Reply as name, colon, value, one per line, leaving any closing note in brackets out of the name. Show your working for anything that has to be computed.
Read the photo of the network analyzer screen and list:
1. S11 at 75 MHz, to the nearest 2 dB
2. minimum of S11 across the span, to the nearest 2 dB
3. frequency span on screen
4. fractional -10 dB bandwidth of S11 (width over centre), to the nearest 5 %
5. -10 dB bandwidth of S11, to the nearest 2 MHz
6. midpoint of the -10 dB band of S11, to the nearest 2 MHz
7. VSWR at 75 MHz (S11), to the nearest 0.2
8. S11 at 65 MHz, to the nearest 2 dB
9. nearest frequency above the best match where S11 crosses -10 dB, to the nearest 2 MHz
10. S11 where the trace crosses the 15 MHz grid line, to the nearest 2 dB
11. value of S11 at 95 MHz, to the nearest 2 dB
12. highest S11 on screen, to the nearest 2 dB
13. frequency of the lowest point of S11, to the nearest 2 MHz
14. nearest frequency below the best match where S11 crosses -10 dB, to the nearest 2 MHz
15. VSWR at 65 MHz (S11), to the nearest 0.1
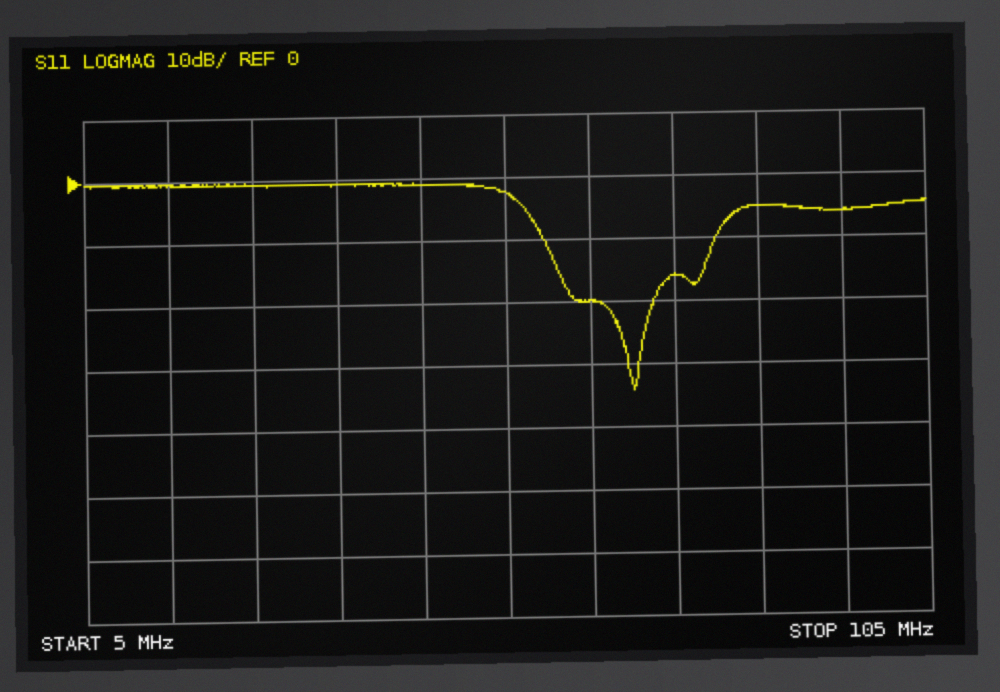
S11 at 75 MHz, to the nearest 2 dB: -16 dB
minimum of S11 across the span, to the nearest 2 dB: -34 dB
frequency span on screen: 100 MHz
fractional -10 dB bandwidth of S11 (width over centre), to the nearest 5 %: 20 MHz / 70 MHz ≈ 28.6 %, so 30 % to the nearest 5 %
-10 dB bandwidth of S11, to the nearest 2 MHz: 80 MHz − 60 MHz = 20 MHz
midpoint of the -10 dB band of S11, to the nearest 2 MHz: 70 MHz
VSWR at 75 MHz (S11), to the nearest 0.2: |Γ| = 10^(-16/20) = 0.1585; VSWR = (1 + 0.1585)/(1 − 0.1585) ≈ 1.4
S11 at 65 MHz, to the nearest 2 dB: -20 dB
nearest frequency above the best match where S11 crosses -10 dB, to the nearest 2 MHz: 80 MHz
S11 where the trace crosses the 15 MHz grid line, to the nearest 2 dB: 0 dB
value of S11 at 95 MHz, to the nearest 2 dB: -6 dB
highest S11 on screen, to the nearest 2 dB: 0 dB
frequency of the lowest point of S11, to the nearest 2 MHz: 70 MHz
nearest frequency below the best match where S11 crosses -10 dB, to the nearest 2 MHz: 60 MHz
VSWR at 65 MHz (S11), to the nearest 0.1: |Γ| = 10^(-20/20) = 0.1000; VSWR = (1 + 0.1000)/(1 − 0.1000) ≈ 1.2
